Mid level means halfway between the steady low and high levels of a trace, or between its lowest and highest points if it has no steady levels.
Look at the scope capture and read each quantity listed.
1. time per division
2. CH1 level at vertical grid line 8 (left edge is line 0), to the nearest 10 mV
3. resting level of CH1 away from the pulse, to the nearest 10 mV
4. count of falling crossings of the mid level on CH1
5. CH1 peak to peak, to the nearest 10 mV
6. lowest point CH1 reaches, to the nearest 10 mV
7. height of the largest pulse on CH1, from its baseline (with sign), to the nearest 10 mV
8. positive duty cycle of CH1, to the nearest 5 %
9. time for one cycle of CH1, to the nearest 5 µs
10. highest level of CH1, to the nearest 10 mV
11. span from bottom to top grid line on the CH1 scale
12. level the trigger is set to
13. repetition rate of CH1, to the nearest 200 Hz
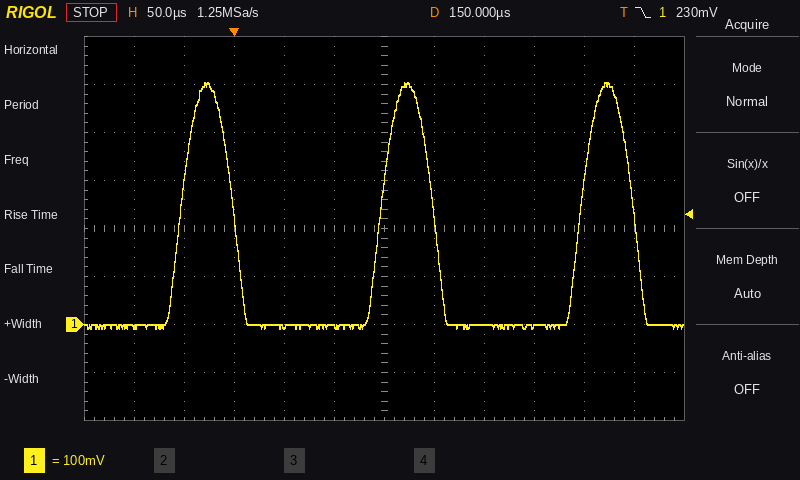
50 µs
0 mV
0 mV
3
510 mV
-10 mV
+500 mV
25 %
200 µs
500 mV
800 mV
230 mV
5.0 kHz
